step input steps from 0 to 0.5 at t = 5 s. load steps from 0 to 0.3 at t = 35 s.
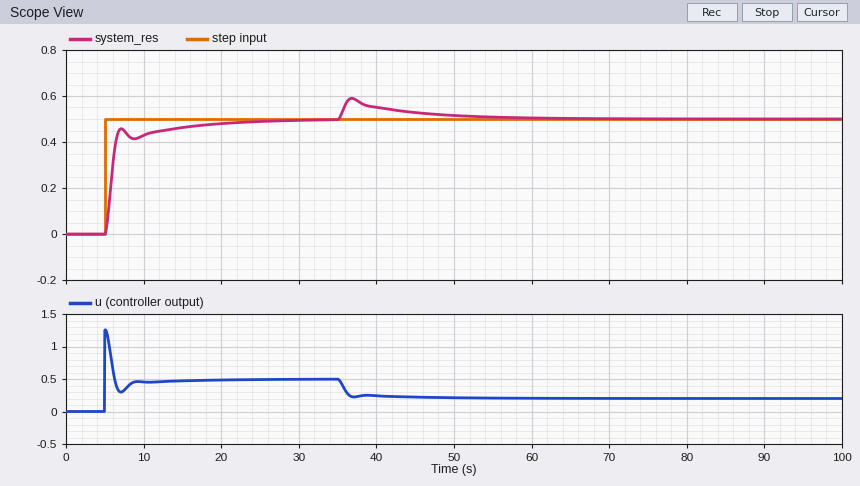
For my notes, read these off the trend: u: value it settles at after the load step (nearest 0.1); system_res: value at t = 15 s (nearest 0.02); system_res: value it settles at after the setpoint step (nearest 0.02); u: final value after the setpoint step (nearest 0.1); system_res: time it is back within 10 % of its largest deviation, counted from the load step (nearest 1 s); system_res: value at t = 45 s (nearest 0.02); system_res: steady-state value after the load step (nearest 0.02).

0.2
0.46
0.50
0.5
19 s
0.52
0.50
